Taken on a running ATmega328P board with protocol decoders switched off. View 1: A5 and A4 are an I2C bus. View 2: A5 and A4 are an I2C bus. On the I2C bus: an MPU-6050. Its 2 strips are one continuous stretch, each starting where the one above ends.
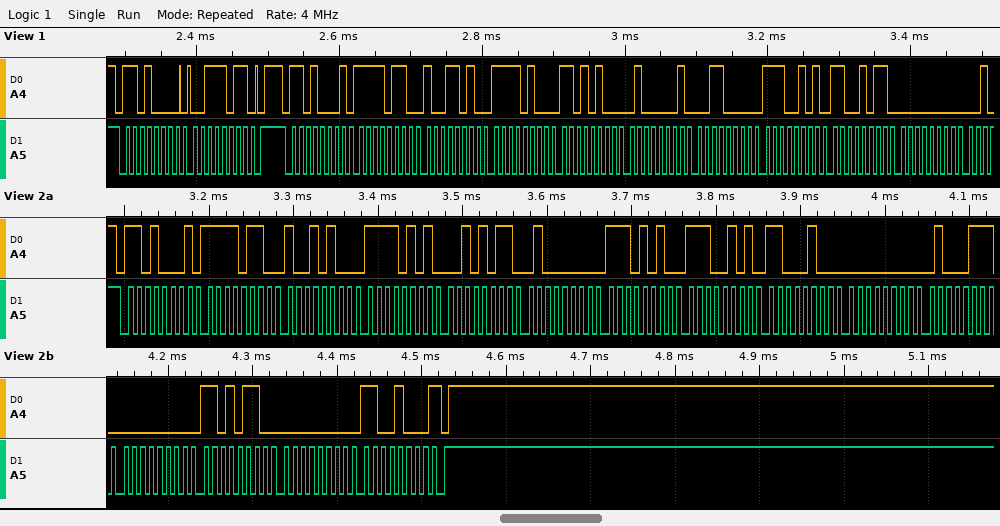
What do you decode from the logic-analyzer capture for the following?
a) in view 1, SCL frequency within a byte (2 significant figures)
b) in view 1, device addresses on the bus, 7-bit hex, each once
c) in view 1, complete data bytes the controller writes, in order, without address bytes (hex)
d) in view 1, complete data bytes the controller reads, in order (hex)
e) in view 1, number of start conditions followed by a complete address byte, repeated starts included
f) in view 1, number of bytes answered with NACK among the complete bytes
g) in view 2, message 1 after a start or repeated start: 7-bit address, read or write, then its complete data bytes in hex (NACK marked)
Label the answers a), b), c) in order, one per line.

a) 100 kHz
b) 0x68
c) 3B
d) F6 9A F4 D4 41 30 E5 CB 00
e) 2
f) 0
g) 0x68 read: F6 94 F5 2B 40 EA E5 C4 00 47 00 D6 00 C8 NACK
